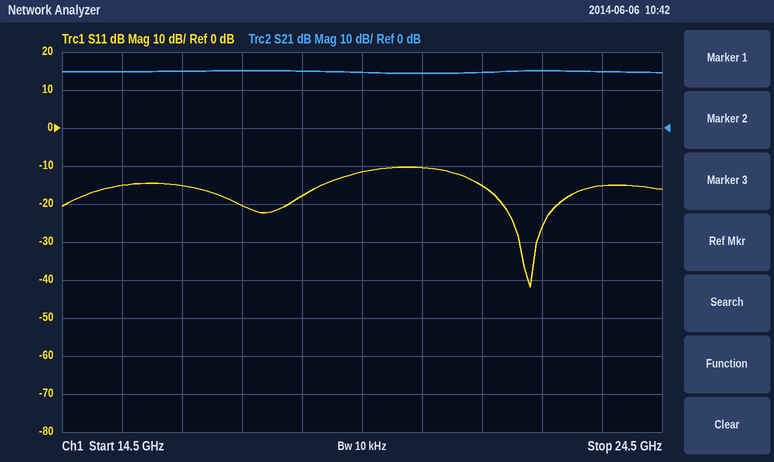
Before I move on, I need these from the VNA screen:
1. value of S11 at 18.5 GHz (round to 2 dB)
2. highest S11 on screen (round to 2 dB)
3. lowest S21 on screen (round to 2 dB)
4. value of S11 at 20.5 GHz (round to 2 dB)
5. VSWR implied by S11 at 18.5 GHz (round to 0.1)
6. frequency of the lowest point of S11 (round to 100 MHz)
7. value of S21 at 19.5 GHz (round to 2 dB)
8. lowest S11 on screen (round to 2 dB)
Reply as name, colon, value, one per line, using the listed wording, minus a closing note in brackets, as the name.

value of S11 at 18.5 GHz: -18 dB
highest S11 on screen: -10 dB
lowest S21 on screen: 14 dB
value of S11 at 20.5 GHz: -10 dB
VSWR implied by S11 at 18.5 GHz: 1.3
frequency of the lowest point of S11: 22.3 GHz
value of S21 at 19.5 GHz: 14 dB
lowest S11 on screen: -42 dB
